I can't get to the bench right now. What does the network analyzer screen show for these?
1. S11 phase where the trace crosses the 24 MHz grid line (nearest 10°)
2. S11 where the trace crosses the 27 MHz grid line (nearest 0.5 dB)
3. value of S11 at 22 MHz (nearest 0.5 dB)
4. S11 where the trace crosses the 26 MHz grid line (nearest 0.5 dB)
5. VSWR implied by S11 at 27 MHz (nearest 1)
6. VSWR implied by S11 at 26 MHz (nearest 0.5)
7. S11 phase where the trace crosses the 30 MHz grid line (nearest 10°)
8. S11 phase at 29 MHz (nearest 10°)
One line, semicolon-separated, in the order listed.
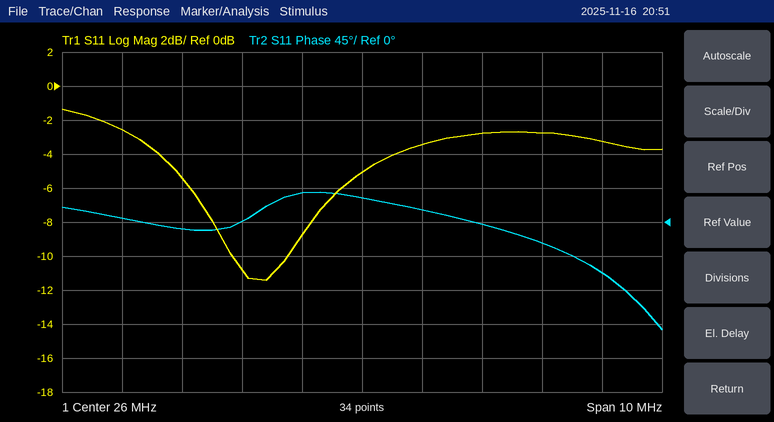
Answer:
0°; -3.5 dB; -2.5 dB; -5.0 dB; 5; 3.5; -70°; -30°
